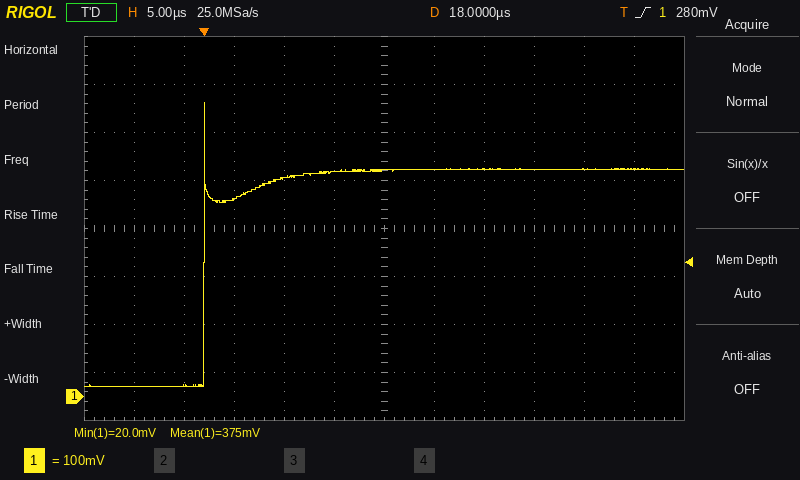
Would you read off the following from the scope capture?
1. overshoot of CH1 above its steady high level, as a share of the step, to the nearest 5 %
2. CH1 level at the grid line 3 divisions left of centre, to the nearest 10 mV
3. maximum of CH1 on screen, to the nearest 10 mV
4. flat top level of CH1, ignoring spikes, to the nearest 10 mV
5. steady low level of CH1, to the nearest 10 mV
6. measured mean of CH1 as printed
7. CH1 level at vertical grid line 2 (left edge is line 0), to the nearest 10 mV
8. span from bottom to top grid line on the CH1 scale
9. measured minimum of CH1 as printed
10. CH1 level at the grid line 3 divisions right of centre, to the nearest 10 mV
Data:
30 %
410 mV
610 mV
470 mV
20 mV
375 mV
20 mV
800 mV
20.0 mV
470 mV
